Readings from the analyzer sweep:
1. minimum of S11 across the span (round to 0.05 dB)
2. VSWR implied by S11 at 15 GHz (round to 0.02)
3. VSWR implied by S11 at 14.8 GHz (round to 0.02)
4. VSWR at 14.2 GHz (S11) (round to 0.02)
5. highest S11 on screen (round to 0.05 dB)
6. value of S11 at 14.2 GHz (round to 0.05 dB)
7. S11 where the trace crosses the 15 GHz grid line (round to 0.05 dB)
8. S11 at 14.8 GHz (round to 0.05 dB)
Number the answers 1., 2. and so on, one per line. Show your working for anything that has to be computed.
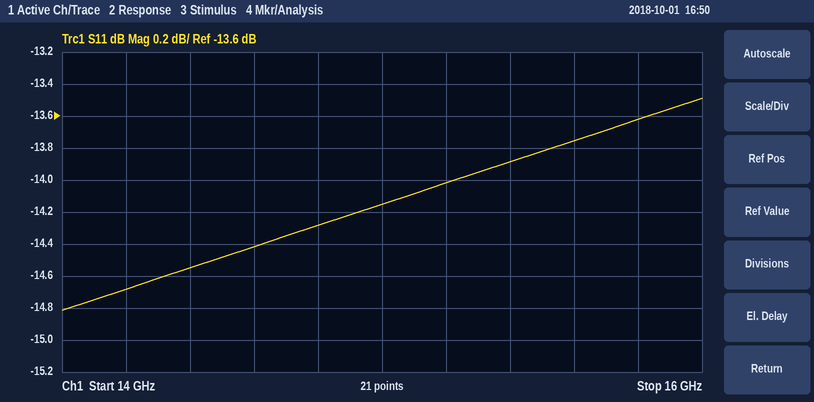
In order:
1. -14.80 dB
2. |Γ| = 10^(-14.15/20) = 0.1961; VSWR = (1 + 0.1961)/(1 − 0.1961) ≈ 1.49, so 1.48 to the nearest 0.02
3. |Γ| = 10^(-14.3/20) = 0.1928; VSWR = (1 + 0.1928)/(1 − 0.1928) ≈ 1.48
4. |Γ| = 10^(-14.7/20) = 0.1841; VSWR = (1 + 0.1841)/(1 − 0.1841) ≈ 1.45, so 1.46 to the nearest 0.02
5. -13.50 dB
6. -14.70 dB
7. -14.15 dB
8. -14.30 dB
